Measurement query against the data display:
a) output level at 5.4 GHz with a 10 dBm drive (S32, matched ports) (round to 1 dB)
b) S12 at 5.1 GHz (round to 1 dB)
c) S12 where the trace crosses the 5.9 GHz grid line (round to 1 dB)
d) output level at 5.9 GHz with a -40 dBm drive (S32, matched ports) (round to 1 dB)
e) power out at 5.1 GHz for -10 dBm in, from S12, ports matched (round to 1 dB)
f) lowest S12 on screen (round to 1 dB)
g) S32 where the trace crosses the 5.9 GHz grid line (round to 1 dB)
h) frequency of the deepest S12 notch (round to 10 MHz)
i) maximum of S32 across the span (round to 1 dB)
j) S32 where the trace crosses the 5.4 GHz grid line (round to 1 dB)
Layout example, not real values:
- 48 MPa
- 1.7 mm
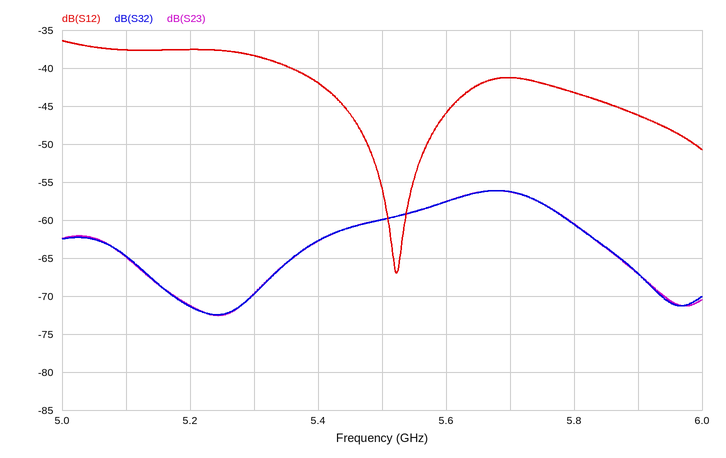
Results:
- -53 dBm
- -38 dB
- -46 dB
- -107 dBm
- -48 dBm
- -67 dB
- -67 dB
- 5.52 GHz
- -56 dB
- -63 dB
